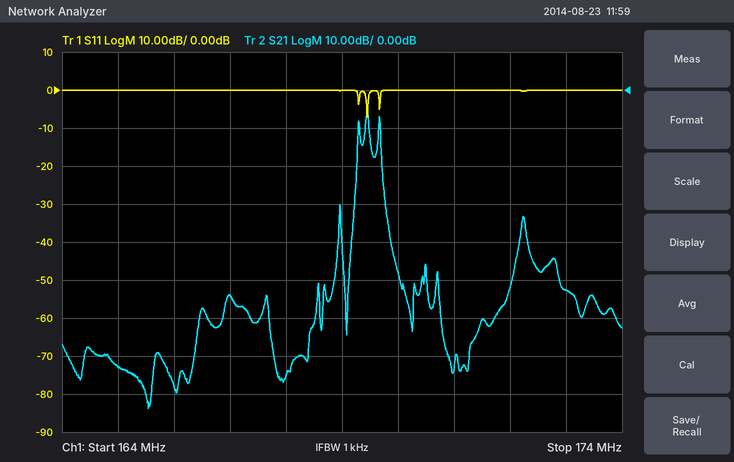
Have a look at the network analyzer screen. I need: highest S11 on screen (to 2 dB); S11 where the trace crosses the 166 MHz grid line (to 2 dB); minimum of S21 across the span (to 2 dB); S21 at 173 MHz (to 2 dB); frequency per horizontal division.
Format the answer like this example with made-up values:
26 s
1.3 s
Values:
0 dB
0 dB
-84 dB
-52 dB
1 MHz
